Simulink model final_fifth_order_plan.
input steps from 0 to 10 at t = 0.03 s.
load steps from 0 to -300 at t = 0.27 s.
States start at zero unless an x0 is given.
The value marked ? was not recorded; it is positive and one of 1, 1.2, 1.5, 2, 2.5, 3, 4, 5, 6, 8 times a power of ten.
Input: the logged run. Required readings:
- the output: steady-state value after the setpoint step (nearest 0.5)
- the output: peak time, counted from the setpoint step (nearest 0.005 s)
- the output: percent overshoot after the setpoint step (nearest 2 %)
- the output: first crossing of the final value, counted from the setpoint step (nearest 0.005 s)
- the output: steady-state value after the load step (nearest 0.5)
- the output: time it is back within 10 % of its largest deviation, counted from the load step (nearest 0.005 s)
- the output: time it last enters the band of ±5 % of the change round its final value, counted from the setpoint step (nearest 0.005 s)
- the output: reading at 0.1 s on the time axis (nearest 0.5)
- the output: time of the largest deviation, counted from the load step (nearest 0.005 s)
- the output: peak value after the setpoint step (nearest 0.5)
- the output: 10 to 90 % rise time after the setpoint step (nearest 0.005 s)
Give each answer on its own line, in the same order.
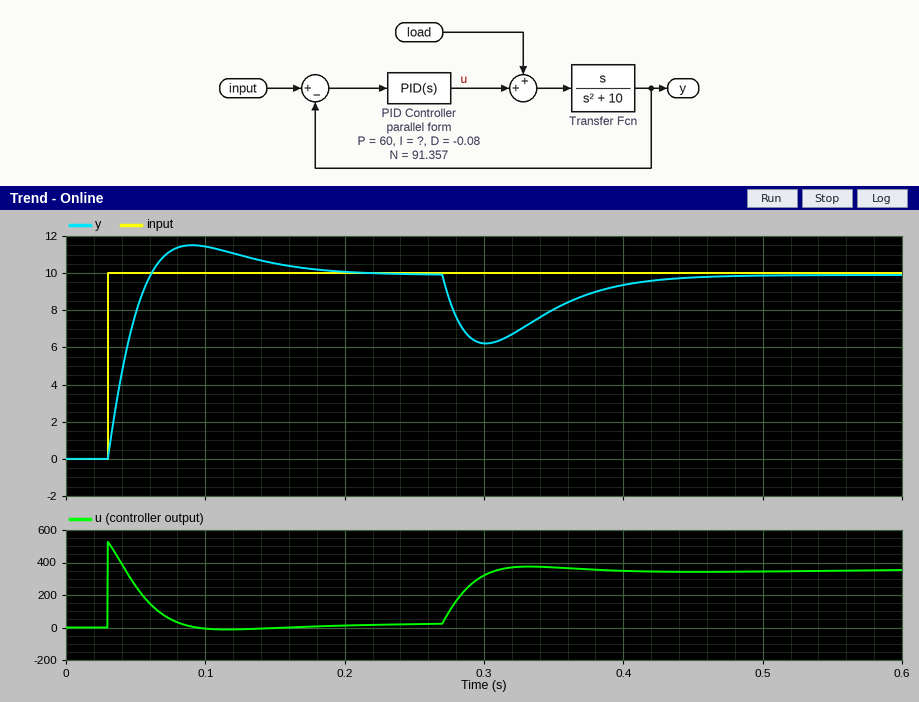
10.0
0.060 s
16 %
0.030 s
10.0
0.145 s
0.130 s
11.5
0.030 s
11.5
0.025 s
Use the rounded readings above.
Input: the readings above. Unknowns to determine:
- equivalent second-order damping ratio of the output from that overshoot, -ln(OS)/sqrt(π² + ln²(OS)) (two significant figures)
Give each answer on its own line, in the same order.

0.50
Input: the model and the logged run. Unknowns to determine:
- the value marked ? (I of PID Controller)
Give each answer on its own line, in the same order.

1000
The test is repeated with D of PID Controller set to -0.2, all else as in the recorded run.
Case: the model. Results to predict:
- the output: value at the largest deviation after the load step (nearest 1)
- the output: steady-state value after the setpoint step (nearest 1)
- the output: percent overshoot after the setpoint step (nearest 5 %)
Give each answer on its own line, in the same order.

6
10
20 %
